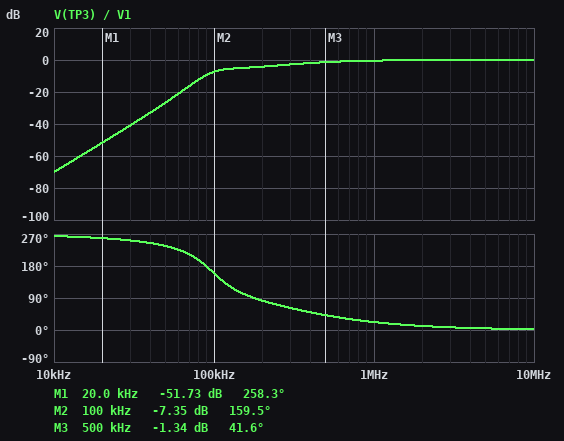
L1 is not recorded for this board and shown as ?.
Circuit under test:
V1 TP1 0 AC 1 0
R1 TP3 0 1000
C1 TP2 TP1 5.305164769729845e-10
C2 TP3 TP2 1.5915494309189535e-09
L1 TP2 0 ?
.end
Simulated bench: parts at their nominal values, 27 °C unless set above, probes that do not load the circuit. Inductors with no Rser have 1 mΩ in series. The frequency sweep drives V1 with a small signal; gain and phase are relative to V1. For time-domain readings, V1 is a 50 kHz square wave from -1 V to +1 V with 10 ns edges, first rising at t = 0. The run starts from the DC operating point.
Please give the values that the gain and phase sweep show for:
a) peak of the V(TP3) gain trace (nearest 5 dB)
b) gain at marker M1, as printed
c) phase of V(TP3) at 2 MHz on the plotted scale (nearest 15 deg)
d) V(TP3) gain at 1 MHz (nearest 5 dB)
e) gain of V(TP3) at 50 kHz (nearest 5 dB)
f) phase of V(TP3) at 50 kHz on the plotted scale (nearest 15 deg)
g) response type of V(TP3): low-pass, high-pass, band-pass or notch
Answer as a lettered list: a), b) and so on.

a) 0 dB
b) -51.73 dB
c) 15 deg
d) 0 dB
e) -25 dB
f) 240 deg
g) high-pass
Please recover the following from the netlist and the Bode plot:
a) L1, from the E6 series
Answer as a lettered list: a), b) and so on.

a) 1.5 mH
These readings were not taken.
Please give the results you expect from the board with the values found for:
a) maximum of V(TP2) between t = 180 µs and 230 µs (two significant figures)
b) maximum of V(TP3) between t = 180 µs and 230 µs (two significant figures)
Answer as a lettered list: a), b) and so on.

a) 1.9 V
b) 2.0 V
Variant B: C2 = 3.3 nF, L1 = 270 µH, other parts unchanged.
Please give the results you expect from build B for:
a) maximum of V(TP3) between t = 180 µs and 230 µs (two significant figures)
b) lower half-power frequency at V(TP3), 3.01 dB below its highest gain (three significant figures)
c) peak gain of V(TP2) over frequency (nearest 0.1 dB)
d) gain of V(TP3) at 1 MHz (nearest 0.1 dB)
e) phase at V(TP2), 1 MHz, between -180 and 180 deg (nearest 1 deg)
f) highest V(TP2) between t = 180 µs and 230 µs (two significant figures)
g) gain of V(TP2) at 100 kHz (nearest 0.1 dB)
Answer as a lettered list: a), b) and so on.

a) 2.0 V
b) 339 kHz
c) 3.3 dB
d) 1.0 dB
e) 20 deg
f) 2.0 V
g) -23.9 dB
